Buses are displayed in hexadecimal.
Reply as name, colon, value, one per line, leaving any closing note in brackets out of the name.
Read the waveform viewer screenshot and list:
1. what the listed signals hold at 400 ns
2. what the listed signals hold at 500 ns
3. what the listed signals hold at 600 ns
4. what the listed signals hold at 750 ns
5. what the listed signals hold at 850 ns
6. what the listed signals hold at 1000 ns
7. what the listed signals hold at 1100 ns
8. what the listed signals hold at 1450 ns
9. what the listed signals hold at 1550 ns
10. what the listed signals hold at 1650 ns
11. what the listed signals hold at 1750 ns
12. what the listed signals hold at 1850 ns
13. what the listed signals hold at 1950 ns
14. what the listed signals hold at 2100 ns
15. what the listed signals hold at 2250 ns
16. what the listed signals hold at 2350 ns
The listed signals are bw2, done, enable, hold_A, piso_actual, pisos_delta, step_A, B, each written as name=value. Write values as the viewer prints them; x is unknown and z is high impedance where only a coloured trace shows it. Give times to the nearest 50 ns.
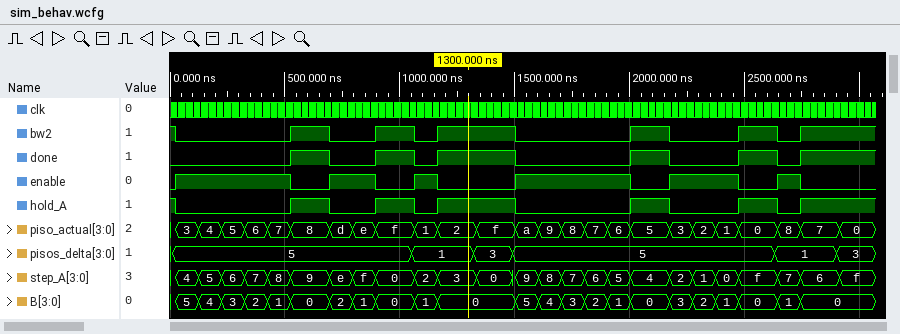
what the listed signals hold at 400 ns: bw2=0, done=0, enable=1, hold_A=0, piso_actual=6, pisos_delta=5, step_A=7, B=2
what the listed signals hold at 500 ns: bw2=0, done=0, enable=1, hold_A=0, piso_actual=7, pisos_delta=5, step_A=8, B=1
what the listed signals hold at 600 ns: bw2=1, done=1, enable=0, hold_A=1, piso_actual=8, pisos_delta=5, step_A=9, B=0
what the listed signals hold at 750 ns: bw2=0, done=0, enable=1, hold_A=0, piso_actual=d, pisos_delta=5, step_A=e, B=2
what the listed signals hold at 850 ns: bw2=0, done=0, enable=1, hold_A=0, piso_actual=e, pisos_delta=5, step_A=f, B=1
what the listed signals hold at 1000 ns: bw2=1, done=1, enable=0, hold_A=1, piso_actual=f, pisos_delta=5, step_A=0, B=0
what the listed signals hold at 1100 ns: bw2=0, done=0, enable=1, hold_A=0, piso_actual=1, pisos_delta=1, step_A=2, B=1
what the listed signals hold at 1450 ns: bw2=1, done=1, enable=0, hold_A=1, piso_actual=f, pisos_delta=3, step_A=0, B=0
what the listed signals hold at 1550 ns: bw2=0, done=0, enable=1, hold_A=0, piso_actual=a, pisos_delta=5, step_A=9, B=5
what the listed signals hold at 1650 ns: bw2=0, done=0, enable=1, hold_A=0, piso_actual=9, pisos_delta=5, step_A=8, B=4
what the listed signals hold at 1750 ns: bw2=0, done=0, enable=1, hold_A=0, piso_actual=8, pisos_delta=5, step_A=7, B=3
what the listed signals hold at 1850 ns: bw2=0, done=0, enable=1, hold_A=0, piso_actual=7, pisos_delta=5, step_A=6, B=2
what the listed signals hold at 1950 ns: bw2=0, done=0, enable=1, hold_A=0, piso_actual=6, pisos_delta=5, step_A=5, B=1
what the listed signals hold at 2100 ns: bw2=1, done=1, enable=0, hold_A=1, piso_actual=5, pisos_delta=5, step_A=4, B=0
what the listed signals hold at 2250 ns: bw2=0, done=0, enable=1, hold_A=0, piso_actual=3, pisos_delta=5, step_A=2, B=3
what the listed signals hold at 2350 ns: bw2=0, done=0, enable=1, hold_A=0, piso_actual=2, pisos_delta=5, step_A=1, B=2
